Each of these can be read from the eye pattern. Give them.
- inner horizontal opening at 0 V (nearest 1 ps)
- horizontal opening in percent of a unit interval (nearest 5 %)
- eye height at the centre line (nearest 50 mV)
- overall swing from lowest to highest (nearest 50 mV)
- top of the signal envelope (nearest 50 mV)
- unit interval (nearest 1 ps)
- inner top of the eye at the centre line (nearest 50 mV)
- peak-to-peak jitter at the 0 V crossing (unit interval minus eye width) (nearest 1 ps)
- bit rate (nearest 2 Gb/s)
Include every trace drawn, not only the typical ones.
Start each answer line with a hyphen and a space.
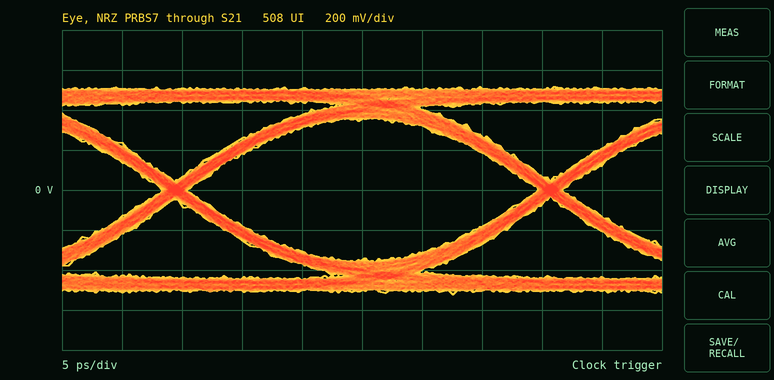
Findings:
- 29 ps
- 95 %
- 700 mV
- 1.05 V
- 500 mV
- 31 ps
- 350 mV
- 2 ps
- 32 Gb/s
